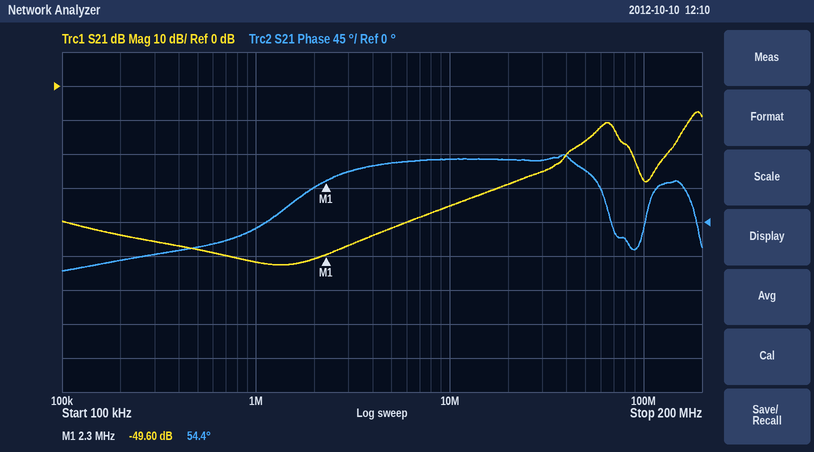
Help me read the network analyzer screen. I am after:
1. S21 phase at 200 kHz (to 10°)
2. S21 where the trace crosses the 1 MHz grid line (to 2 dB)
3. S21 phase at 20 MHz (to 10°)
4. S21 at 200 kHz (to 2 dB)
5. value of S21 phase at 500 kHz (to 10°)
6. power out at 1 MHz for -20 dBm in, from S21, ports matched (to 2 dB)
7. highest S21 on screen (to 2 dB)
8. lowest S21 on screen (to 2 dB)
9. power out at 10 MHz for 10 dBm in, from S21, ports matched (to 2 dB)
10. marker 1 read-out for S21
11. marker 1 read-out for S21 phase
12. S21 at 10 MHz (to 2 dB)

-50°
-52 dB
80°
-44 dB
-30°
-72 dBm
-8 dB
-52 dB
-26 dBm
-49.60 dB
54.4°
-36 dB
